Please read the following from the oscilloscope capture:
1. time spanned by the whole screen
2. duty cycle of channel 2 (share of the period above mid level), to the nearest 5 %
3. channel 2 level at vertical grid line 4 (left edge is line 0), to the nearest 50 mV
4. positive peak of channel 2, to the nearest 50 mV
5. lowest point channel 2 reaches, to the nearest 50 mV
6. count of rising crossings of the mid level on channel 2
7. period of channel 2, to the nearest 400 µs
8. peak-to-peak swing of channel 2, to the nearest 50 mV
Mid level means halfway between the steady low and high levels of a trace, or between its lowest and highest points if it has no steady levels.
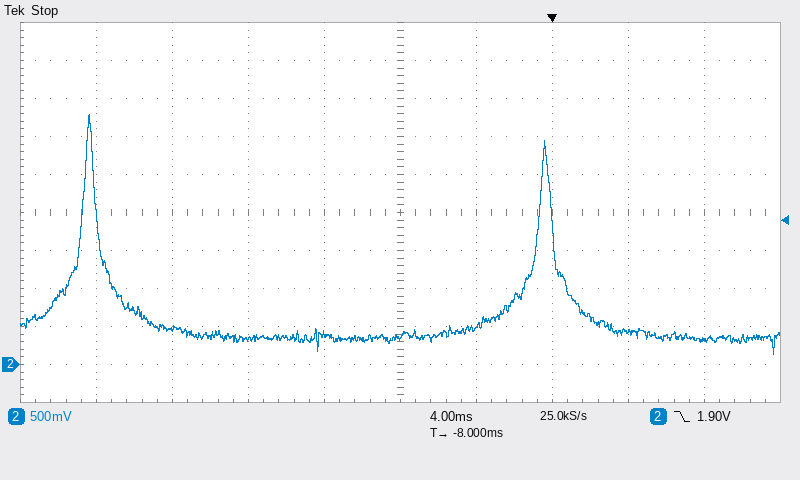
40 ms
5 %
400 mV
3.30 V
150 mV
2
24.0 ms
3.15 V
